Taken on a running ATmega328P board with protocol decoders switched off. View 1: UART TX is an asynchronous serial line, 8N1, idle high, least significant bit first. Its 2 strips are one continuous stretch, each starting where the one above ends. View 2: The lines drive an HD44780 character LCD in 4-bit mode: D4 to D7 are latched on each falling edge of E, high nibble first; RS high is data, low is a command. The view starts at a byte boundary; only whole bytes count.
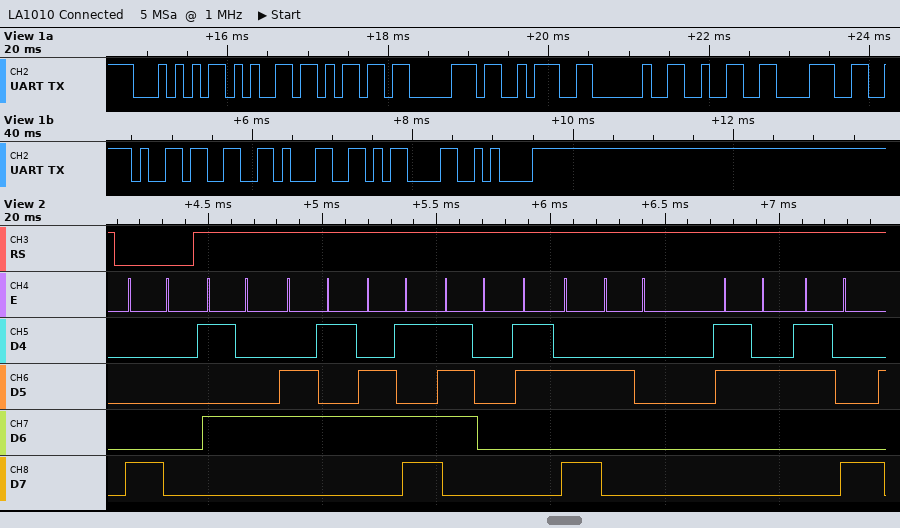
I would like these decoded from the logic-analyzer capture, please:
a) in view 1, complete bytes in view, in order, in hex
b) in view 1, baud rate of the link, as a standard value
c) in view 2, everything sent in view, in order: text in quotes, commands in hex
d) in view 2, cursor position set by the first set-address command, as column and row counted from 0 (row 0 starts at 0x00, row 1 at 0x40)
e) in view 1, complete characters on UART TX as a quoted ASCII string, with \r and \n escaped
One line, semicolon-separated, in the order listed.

54 65 6D 70 3A 20 32 38 2E 33 31 0D 0A; 9600 baud; 0x80 "Temp: 28"; column 0, row 0; "Temp: 28.31\r\n"
